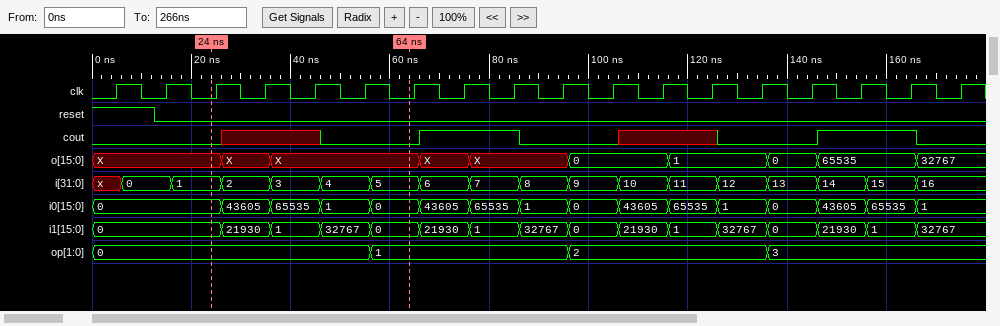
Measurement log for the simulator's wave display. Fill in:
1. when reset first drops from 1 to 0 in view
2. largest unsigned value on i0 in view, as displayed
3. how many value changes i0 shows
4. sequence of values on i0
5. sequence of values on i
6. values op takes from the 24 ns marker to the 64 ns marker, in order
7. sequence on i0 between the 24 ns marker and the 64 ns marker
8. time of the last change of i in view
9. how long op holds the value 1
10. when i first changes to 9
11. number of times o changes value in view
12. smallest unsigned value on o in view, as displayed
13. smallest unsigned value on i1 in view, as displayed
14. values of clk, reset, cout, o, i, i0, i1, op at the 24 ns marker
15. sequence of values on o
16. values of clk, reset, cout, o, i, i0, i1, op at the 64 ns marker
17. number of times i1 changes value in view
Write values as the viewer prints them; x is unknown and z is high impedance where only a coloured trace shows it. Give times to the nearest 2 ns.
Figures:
12 ns
65535
15
0, 43605, 65535, 1, 0, 43605, 65535, 1, 0, 43605, 65535, 1, 0, 43605, 65535, 1
x, 0, 1, 2, 3, 4, 5, 6, 7, 8, 9, 10, 11, 12, 13, 14, 15, 16
0, 1
0, 43605, 65535, 1, 0
166 ns
40 ns
96 ns
9
0
0
clk=0, reset=0, cout=0, o=X, i=1, i0=0, i1=0, op=0
X, X, X, X, X, 0, 1, 0, 65535, 32767
clk=0, reset=0, cout=0, o=X, i=5, i0=0, i1=0, op=1
15
